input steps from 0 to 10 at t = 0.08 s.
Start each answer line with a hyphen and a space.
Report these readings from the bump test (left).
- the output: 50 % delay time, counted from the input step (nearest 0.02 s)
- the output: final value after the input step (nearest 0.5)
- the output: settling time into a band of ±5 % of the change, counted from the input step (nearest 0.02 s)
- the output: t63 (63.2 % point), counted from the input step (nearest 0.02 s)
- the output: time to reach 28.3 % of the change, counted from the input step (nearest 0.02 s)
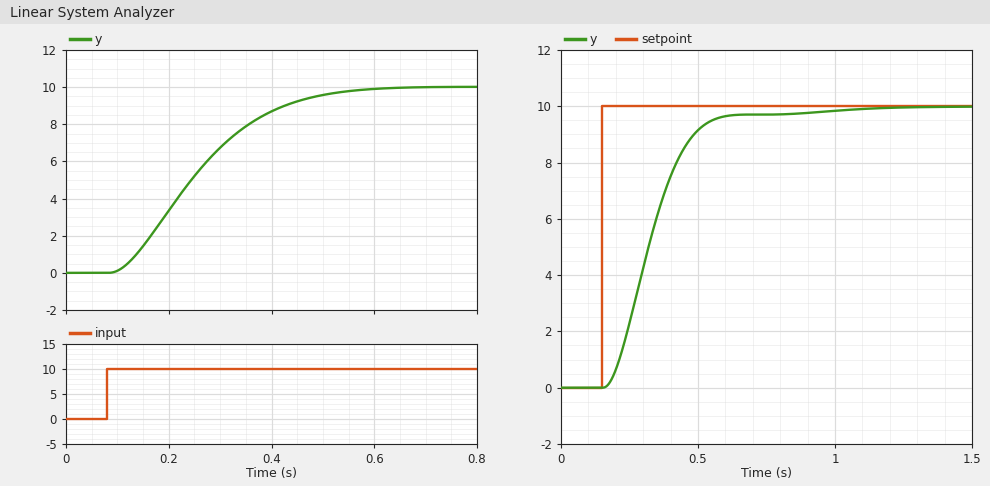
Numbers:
- 0.16 s
- 10.0
- 0.40 s
- 0.20 s
- 0.10 s
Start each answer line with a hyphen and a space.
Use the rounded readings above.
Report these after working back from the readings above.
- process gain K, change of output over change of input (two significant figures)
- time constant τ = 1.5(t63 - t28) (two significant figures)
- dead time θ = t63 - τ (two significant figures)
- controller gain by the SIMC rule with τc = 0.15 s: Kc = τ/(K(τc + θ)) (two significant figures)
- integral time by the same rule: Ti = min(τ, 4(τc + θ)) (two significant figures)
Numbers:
- 1.0
- 0.15 s
- 0.050 s
- 0.75
- 0.15 s
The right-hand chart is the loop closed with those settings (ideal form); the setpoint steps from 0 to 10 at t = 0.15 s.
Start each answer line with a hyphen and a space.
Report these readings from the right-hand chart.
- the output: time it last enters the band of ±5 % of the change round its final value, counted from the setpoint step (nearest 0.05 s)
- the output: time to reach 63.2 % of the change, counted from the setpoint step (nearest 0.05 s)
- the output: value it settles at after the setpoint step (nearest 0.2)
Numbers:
- 0.40 s
- 0.20 s
- 10.0
